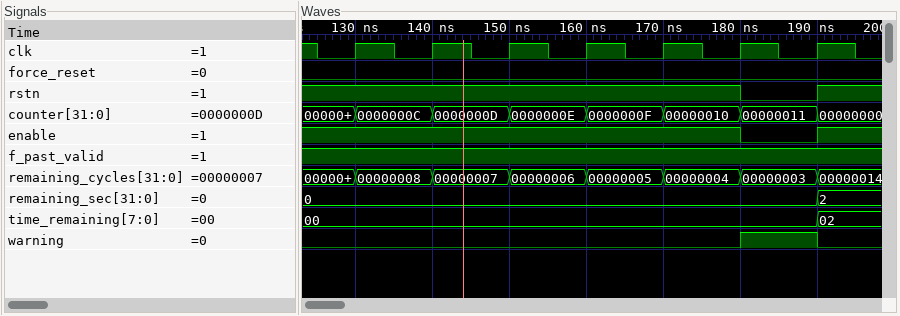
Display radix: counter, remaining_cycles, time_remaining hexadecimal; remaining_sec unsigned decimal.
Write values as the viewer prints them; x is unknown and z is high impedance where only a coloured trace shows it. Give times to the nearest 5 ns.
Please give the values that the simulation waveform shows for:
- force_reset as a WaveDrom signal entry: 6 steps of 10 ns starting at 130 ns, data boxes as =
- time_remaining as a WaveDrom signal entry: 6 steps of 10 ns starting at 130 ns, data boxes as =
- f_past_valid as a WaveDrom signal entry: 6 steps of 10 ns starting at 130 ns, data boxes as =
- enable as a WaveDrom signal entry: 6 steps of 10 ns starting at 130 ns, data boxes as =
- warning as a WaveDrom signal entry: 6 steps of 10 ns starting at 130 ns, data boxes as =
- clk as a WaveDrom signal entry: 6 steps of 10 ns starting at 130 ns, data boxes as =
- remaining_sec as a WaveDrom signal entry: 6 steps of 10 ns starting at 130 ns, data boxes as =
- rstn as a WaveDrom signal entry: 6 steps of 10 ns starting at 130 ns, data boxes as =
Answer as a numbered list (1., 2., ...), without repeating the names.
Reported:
1. {name: 'force_reset', wave: '0.....'}
2. {name: 'time_remaining', wave: '=.....', data: '00'}
3. {name: 'f_past_valid', wave: '1.....'}
4. {name: 'enable', wave: '1....0'}
5. {name: 'warning', wave: '0....1'}
6. {name: 'clk', wave: 'p.....'}
7. {name: 'remaining_sec', wave: '=.....', data: '0'}
8. {name: 'rstn', wave: '1....0'}
